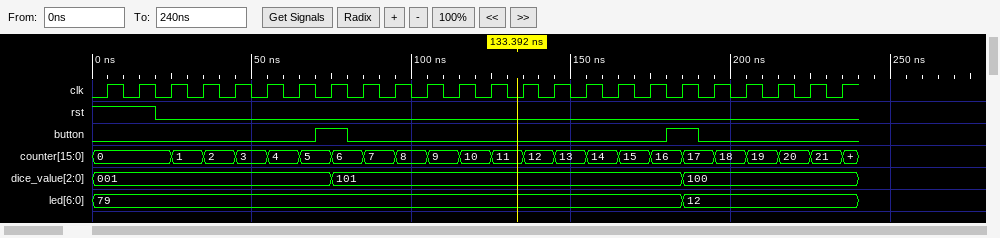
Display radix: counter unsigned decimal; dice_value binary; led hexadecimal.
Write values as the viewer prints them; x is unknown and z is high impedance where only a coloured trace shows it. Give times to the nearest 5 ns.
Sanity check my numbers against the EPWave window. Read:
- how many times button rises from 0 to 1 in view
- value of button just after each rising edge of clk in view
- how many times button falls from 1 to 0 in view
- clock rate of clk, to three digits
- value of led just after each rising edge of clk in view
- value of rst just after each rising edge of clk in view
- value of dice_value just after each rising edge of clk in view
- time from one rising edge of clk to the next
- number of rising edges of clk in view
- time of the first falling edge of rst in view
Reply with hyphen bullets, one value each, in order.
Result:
- 2
- 0 0 0 0 0 0 0 1 0 0 0 0 0 0 0 0 0 0 1 0 0 0 0 0
- 2
- 100 MHz
- 79, 79, 79, 79, 79, 79, 79, 79, 79, 79, 79, 79, 79, 79, 79, 79, 79, 79, 12, 12, 12, 12, 12, 12
- 1 1 0 0 0 0 0 0 0 0 0 0 0 0 0 0 0 0 0 0 0 0 0 0
- 001, 001, 001, 001, 001, 001, 001, 101, 101, 101, 101, 101, 101, 101, 101, 101, 101, 101, 100, 100, 100, 100, 100, 100
- 10 ns
- 24
- 20 ns
